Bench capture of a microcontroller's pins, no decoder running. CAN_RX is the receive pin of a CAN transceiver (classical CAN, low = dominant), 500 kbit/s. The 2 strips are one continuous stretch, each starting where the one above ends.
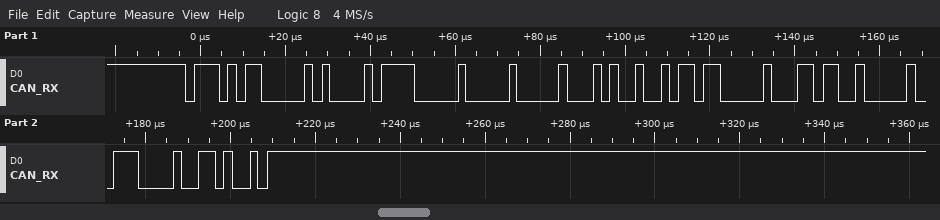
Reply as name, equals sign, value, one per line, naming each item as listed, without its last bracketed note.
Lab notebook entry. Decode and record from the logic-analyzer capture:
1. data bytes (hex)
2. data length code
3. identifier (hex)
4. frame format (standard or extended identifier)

data bytes = 5E 00 00 52 5B 00 D9 01
data length code = 8
identifier = 0x758
frame format = standard
